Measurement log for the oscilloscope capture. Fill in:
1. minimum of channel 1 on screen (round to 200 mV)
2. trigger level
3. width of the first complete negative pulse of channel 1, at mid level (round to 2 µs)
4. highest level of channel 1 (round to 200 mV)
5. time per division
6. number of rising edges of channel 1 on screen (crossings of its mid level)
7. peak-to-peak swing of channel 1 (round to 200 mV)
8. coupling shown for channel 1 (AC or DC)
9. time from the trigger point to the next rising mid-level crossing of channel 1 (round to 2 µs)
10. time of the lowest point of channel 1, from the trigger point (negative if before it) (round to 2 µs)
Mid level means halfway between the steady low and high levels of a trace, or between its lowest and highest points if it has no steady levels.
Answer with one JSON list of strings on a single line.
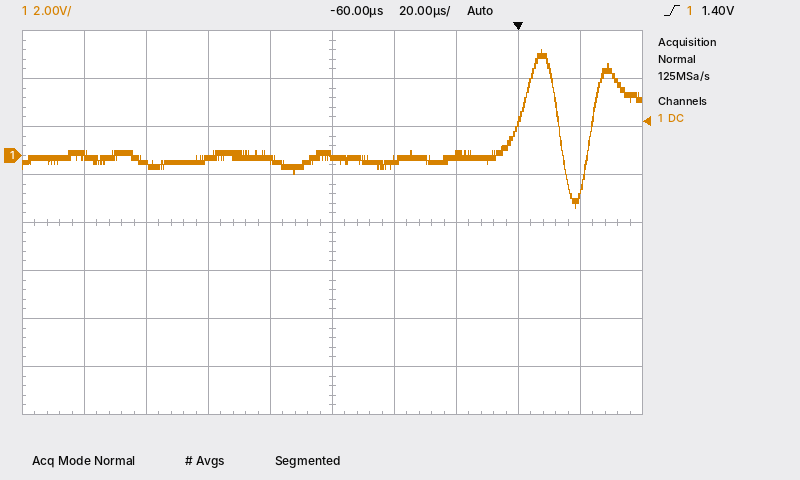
["-2.2 V", "1.40 V", "10 µs", "4.4 V", "20 µs", "2", "6.6 V", "DC", "24 µs", "+18 µs"]
